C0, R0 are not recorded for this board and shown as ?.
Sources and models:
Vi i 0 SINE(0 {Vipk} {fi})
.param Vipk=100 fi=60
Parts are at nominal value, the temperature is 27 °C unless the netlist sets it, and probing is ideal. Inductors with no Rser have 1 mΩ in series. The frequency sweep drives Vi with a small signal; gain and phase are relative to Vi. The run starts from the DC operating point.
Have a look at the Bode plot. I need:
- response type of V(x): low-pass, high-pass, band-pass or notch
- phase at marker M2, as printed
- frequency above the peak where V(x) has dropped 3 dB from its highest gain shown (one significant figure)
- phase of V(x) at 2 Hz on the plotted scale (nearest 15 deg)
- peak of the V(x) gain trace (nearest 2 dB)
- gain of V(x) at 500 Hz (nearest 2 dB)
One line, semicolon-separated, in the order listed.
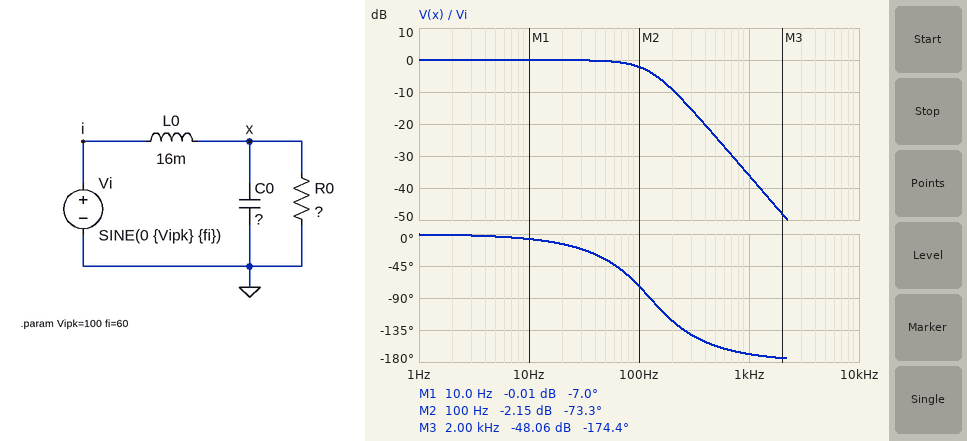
low-pass; -73.3 deg; 100 Hz; 0 deg; 0 dB; -24 dB
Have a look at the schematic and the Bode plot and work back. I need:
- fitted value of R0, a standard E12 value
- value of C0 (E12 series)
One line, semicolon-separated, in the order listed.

8.2 Ω; 100 µF
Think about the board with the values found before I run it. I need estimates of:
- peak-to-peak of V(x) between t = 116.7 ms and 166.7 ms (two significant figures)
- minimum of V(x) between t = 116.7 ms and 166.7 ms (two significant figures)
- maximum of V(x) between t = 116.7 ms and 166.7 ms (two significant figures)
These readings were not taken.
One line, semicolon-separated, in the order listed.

190 V; -94 V; 94 V
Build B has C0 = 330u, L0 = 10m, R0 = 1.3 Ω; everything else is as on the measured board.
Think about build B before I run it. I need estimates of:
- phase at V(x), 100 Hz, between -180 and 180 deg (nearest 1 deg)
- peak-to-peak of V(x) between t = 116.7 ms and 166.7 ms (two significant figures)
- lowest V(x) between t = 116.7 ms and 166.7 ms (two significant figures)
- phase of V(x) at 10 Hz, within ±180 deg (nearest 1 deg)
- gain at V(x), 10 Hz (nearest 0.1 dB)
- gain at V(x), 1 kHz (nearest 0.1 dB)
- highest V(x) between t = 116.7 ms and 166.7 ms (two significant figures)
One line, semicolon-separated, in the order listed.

-94 deg; 68 V; -34 V; -26 deg; -0.8 dB; -42.8 dB; 34 V
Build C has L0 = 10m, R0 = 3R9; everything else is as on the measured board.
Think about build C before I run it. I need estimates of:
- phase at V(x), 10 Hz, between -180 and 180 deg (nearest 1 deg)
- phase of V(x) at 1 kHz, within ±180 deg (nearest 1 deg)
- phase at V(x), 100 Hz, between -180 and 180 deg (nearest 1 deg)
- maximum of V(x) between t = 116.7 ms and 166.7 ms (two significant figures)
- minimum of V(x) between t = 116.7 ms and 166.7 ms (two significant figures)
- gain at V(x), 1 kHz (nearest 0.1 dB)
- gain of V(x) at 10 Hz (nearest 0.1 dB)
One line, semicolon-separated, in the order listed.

-9 deg; -157 deg; -69 deg; 77 V; -77 V; -32.4 dB; -0.1 dB
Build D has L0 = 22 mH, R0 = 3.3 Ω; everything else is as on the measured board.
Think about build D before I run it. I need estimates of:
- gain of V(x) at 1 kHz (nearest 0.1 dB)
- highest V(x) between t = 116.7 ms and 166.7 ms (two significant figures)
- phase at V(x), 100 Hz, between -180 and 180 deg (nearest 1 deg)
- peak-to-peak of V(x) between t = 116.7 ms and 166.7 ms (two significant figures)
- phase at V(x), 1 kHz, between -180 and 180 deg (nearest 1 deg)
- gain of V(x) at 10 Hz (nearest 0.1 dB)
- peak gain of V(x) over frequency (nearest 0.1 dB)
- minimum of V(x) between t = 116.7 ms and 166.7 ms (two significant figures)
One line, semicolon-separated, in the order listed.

-39.6 dB; 38 V; -88 deg; 77 V; -154 deg; -0.6 dB; 0 dB; -38 V
